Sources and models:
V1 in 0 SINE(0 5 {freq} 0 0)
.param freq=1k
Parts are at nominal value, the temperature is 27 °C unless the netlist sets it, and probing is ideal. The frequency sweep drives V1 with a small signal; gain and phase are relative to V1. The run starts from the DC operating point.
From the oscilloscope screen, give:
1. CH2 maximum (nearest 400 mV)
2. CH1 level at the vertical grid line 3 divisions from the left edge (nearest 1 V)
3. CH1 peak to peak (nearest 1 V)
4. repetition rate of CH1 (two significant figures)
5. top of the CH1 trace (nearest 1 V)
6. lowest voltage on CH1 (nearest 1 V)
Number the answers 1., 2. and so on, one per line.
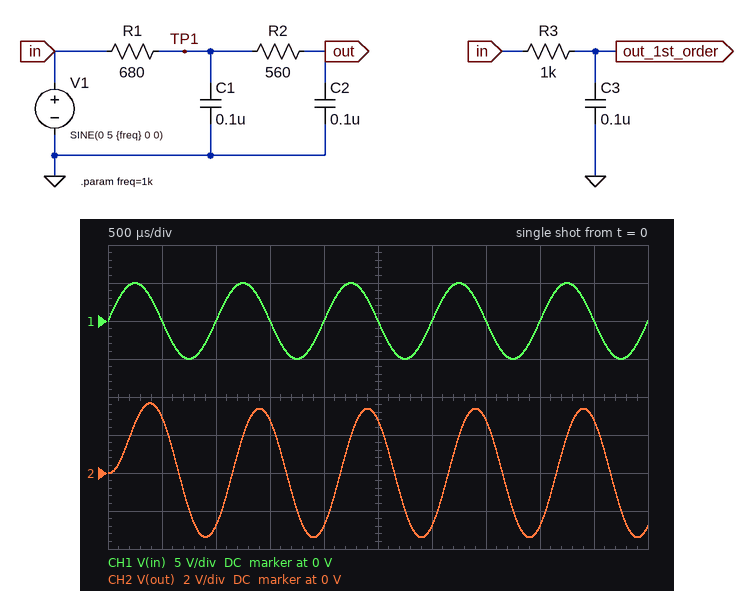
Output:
1. 3.6 V
2. 0 V
3. 10 V
4. 1.0 kHz
5. 5 V
6. -5 V
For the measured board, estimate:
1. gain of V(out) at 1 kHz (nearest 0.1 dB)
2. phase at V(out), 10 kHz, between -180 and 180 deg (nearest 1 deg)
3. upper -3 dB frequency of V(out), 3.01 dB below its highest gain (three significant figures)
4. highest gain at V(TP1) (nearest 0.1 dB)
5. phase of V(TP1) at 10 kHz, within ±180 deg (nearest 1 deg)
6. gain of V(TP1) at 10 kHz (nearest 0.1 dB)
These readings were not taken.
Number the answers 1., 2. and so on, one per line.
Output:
1. -3.4 dB
2. -139 deg
3. 923 Hz
4. 0 dB
5. -65 deg
6. -14.1 dB
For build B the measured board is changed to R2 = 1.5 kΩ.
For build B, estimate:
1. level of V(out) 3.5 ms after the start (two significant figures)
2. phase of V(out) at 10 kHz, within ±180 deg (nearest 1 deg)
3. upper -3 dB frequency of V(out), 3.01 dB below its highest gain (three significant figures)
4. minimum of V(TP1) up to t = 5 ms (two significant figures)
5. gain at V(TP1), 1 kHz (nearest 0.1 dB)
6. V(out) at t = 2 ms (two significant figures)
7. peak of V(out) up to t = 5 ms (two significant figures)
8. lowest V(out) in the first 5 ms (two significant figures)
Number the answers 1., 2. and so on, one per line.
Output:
1. 2.5 V
2. -155 deg
3. 634 Hz
4. -3.6 V
5. -2.8 dB
6. -2.5 V
7. 3.1 V
8. -2.6 V
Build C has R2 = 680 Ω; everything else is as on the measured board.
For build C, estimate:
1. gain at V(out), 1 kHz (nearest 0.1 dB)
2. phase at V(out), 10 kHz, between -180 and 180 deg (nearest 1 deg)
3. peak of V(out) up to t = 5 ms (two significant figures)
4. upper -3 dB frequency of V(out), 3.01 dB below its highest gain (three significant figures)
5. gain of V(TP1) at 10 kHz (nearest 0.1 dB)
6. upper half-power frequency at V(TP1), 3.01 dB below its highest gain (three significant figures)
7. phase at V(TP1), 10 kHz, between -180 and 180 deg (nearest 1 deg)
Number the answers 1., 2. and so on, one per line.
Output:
1. -3.6 dB
2. -143 deg
3. 3.6 V
4. 876 Hz
5. -13.8 dB
6. 1.03 kHz
7. -67 deg
